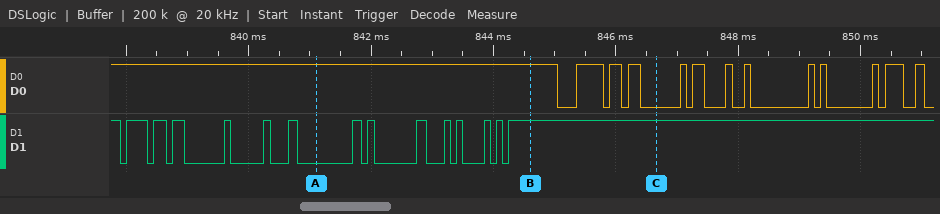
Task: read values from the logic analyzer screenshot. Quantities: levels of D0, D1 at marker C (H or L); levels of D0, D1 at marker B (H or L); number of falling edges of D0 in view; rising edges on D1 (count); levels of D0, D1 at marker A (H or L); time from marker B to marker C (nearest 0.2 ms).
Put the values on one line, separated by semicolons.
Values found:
D0=L, D1=H; D0=H, D1=H; 13; 14; D0=H, D1=L; 2 ms
